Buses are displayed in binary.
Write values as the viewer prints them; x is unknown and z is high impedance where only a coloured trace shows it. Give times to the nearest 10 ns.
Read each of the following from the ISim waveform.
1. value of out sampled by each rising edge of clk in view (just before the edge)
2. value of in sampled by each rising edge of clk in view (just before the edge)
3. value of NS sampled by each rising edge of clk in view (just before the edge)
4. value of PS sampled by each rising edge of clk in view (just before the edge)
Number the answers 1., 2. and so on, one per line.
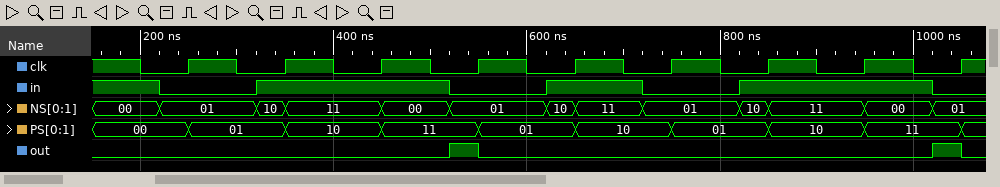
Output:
1. 0 0 0 1 0 0 0 0 1
2. 0 1 1 0 1 0 1 1 0
3. 01, 10, 11, 01, 10, 01, 10, 11, 01
4. 00, 01, 10, 11, 01, 10, 01, 10, 11
